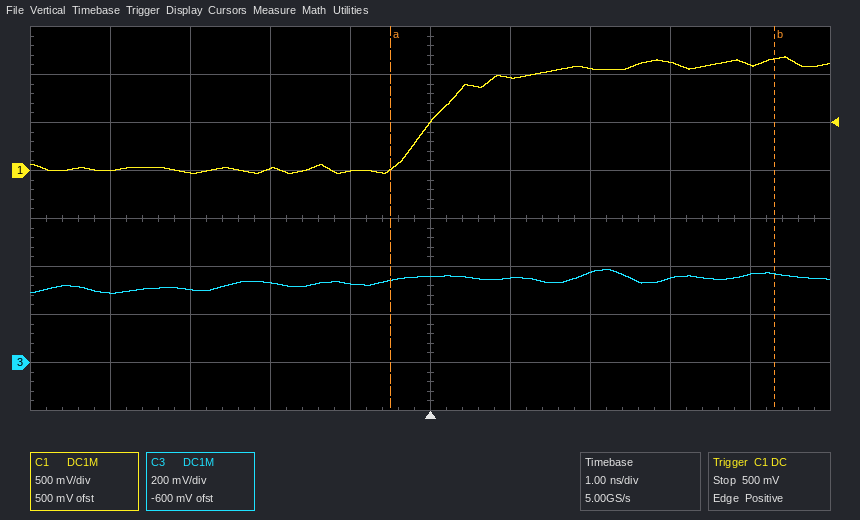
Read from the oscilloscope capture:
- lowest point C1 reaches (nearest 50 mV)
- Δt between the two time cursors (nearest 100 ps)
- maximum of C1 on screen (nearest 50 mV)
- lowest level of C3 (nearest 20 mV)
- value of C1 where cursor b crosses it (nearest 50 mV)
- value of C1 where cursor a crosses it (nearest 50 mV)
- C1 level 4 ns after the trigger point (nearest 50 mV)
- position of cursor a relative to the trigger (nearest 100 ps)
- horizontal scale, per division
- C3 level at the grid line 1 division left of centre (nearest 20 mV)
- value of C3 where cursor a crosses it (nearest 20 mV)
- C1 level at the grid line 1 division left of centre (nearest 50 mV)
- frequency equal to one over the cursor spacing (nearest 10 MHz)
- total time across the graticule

-50 mV
4.8 ns
1.20 V
280 mV
1.15 V
0 mV
1.10 V
-500 ps
1 ns
320 mV
340 mV
0 mV
210 MHz
10 ns
